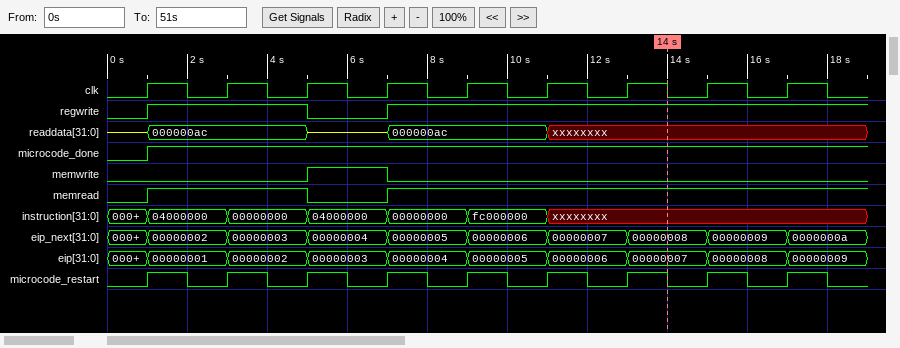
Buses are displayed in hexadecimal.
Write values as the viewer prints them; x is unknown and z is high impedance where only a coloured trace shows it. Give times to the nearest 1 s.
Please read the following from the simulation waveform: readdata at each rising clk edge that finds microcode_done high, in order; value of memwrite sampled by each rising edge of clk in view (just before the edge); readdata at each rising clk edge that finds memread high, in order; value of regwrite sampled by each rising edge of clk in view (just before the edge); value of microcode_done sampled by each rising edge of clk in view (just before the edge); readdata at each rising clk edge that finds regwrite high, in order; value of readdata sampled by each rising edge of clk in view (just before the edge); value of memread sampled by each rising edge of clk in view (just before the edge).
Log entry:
000000ac, 000000ac, z, 000000ac, 000000ac, xxxxxxxx, xxxxxxxx, xxxxxxxx
0 0 0 1 0 0 0 0 0
000000ac, 000000ac, 000000ac, 000000ac, xxxxxxxx, xxxxxxxx, xxxxxxxx
0 1 1 0 1 1 1 1 1
0 1 1 1 1 1 1 1 1
000000ac, 000000ac, 000000ac, 000000ac, xxxxxxxx, xxxxxxxx, xxxxxxxx
z, 000000ac, 000000ac, z, 000000ac, 000000ac, xxxxxxxx, xxxxxxxx, xxxxxxxx
0 1 1 0 1 1 1 1 1
